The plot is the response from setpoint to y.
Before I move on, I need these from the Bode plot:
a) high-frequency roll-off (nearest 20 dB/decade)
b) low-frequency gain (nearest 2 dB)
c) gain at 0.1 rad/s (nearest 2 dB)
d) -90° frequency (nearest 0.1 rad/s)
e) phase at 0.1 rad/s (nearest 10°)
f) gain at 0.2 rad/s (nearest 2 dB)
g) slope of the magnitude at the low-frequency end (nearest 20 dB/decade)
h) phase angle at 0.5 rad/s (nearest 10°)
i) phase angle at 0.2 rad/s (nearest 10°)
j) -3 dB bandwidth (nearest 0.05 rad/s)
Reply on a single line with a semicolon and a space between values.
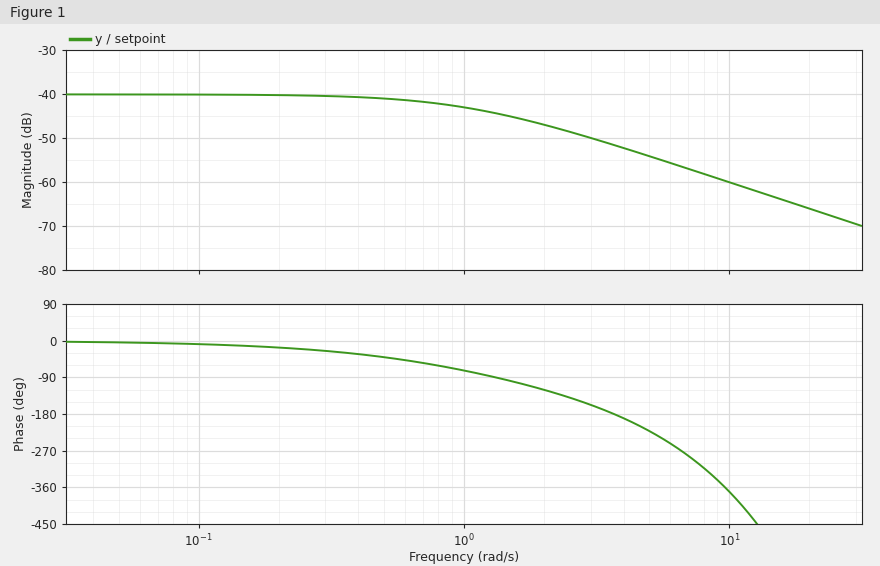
-20 dB/decade; -40 dB; -40 dB; 1.3 rad/s; -10°; -40 dB; 0 dB/decade; -40°; -20°; 1.00 rad/s
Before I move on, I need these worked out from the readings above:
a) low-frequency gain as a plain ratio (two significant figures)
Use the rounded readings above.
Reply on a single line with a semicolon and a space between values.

0.010
